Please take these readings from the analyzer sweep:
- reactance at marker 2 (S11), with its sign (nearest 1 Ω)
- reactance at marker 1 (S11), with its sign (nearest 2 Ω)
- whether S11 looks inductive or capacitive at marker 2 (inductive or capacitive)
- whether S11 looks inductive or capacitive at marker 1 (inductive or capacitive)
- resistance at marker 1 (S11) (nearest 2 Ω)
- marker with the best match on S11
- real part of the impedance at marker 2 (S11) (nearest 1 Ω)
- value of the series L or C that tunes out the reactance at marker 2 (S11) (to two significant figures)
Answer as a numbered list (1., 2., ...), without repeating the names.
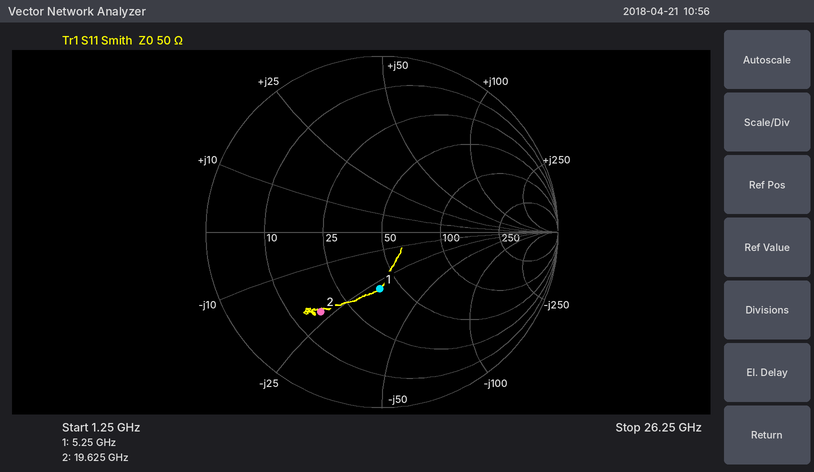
1. -22 Ω
2. -28 Ω
3. capacitive
4. capacitive
5. 40 Ω
6. marker 1
7. 17 Ω
8. 180 pH
